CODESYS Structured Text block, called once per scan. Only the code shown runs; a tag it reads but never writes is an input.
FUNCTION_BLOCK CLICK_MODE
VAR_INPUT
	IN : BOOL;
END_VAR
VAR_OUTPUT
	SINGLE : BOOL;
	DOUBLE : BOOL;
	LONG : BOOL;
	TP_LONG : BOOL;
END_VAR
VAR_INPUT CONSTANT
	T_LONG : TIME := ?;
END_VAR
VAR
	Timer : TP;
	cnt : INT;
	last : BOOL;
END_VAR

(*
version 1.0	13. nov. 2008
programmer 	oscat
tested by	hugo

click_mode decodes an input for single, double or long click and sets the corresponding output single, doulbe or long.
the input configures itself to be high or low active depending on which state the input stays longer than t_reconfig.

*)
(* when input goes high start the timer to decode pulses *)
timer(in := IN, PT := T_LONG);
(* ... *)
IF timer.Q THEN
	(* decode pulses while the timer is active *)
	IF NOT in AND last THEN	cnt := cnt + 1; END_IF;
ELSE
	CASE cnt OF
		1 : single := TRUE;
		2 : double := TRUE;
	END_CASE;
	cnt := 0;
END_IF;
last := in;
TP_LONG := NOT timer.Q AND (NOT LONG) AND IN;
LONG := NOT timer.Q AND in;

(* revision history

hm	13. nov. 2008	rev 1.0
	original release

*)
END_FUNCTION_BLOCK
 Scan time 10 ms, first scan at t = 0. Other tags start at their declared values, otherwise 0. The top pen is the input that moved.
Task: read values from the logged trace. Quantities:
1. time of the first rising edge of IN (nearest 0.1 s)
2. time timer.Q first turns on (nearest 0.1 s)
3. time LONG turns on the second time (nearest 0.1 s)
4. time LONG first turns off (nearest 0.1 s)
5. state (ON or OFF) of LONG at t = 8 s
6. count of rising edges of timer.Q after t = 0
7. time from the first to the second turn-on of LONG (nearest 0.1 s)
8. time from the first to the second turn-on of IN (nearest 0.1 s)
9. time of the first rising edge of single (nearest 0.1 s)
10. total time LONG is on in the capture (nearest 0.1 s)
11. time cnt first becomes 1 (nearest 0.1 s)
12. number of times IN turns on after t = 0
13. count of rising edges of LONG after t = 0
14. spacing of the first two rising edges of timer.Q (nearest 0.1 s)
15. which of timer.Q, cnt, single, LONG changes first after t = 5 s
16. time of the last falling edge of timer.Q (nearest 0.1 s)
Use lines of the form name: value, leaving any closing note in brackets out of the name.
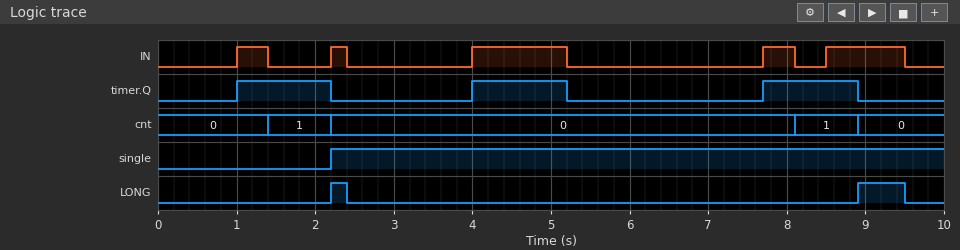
time of the first rising edge of IN: 1.0 s
time timer.Q first turns on: 1.0 s
time LONG turns on the second time: 8.9 s
time LONG first turns off: 2.4 s
state (ON or OFF) of LONG at t = 8 s: OFF
count of rising edges of timer.Q after t = 0: 3
time from the first to the second turn-on of LONG: 6.7 s
time from the first to the second turn-on of IN: 1.2 s
time of the first rising edge of single: 2.2 s
total time LONG is on in the capture: 0.8 s
time cnt first becomes 1: 1.4 s
number of times IN turns on after t = 0: 5
count of rising edges of LONG after t = 0: 2
spacing of the first two rising edges of timer.Q: 3.0 s
which of timer.Q, cnt, single, LONG changes first after t = 5 s: timer.Q
time of the last falling edge of timer.Q: 8.9 s
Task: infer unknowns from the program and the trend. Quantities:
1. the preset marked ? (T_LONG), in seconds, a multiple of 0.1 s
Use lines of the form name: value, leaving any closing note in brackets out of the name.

the preset marked ? (T_LONG), in seconds, a multiple of 0.1 s: 1.2 s
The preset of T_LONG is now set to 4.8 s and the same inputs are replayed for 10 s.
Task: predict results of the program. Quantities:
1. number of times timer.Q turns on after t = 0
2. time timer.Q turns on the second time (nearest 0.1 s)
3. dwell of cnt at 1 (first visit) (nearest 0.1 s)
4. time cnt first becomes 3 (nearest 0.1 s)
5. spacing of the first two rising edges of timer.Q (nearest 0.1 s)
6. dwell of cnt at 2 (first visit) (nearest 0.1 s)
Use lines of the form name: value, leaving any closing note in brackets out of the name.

number of times timer.Q turns on after t = 0: 2
time timer.Q turns on the second time: 7.7 s
dwell of cnt at 1 (first visit): 1.0 s
time cnt first becomes 3: 5.2 s
spacing of the first two rising edges of timer.Q: 6.7 s
dwell of cnt at 2 (first visit): 2.8 s
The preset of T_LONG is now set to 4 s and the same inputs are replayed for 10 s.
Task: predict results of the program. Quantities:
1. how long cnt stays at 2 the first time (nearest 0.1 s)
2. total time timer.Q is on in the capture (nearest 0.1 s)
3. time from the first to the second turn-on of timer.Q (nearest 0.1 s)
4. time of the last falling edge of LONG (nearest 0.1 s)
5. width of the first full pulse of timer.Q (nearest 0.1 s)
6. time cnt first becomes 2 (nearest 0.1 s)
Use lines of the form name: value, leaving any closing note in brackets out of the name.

how long cnt stays at 2 the first time: 2.6 s
total time timer.Q is on in the capture: 6.3 s
time from the first to the second turn-on of timer.Q: 6.7 s
time of the last falling edge of LONG: 5.2 s
width of the first full pulse of timer.Q: 4.0 s
time cnt first becomes 2: 2.4 s
